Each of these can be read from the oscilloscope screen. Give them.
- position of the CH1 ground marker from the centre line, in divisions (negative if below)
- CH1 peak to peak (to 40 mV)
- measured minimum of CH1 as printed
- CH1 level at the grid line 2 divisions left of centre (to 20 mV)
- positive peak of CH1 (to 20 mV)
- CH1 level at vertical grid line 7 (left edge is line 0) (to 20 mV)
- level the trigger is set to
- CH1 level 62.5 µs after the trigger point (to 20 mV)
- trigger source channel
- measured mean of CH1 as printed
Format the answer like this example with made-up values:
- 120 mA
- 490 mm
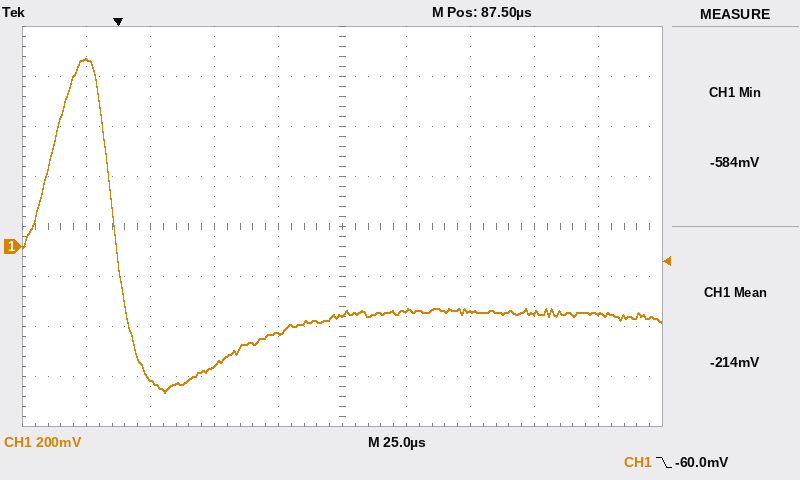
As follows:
- -0.4 div
- 1.32 V
- -584 mV
- -480 mV
- 760 mV
- -260 mV
- -60.0 mV
- -340 mV
- CH1
- -214 mV
